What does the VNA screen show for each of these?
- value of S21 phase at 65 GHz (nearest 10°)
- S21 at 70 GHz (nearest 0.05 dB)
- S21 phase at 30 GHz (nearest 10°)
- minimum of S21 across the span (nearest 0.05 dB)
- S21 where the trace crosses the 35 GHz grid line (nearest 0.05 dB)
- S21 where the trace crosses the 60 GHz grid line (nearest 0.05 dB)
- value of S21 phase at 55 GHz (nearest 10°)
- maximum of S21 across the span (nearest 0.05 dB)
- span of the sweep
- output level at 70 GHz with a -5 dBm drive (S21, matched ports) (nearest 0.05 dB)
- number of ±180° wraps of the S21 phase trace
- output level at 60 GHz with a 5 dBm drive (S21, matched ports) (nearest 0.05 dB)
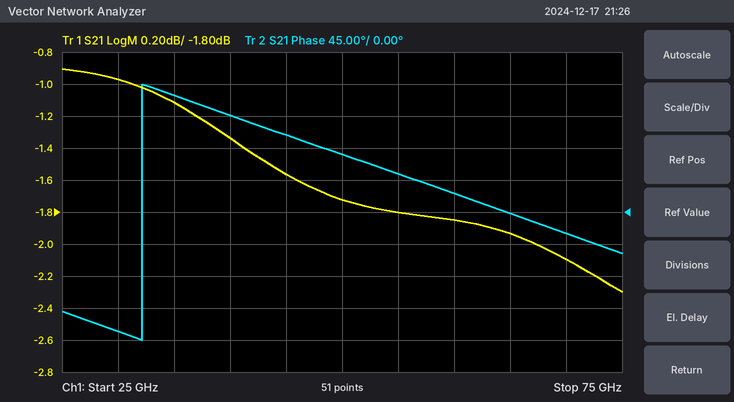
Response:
0°
-2.10 dB
-170°
-2.30 dB
-1.10 dB
-1.85 dB
50°
-0.90 dB
50 GHz
-7.10 dBm
1
3.15 dBm
